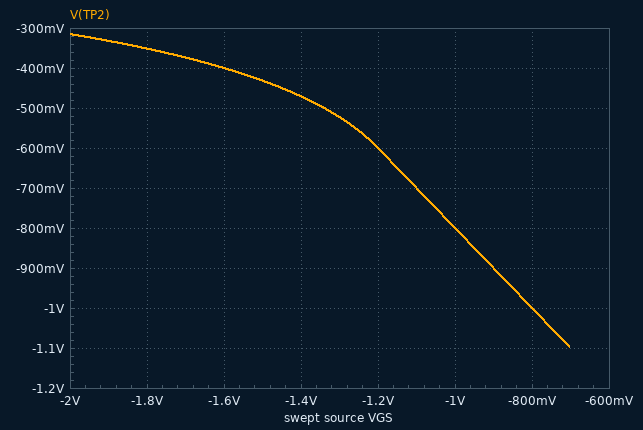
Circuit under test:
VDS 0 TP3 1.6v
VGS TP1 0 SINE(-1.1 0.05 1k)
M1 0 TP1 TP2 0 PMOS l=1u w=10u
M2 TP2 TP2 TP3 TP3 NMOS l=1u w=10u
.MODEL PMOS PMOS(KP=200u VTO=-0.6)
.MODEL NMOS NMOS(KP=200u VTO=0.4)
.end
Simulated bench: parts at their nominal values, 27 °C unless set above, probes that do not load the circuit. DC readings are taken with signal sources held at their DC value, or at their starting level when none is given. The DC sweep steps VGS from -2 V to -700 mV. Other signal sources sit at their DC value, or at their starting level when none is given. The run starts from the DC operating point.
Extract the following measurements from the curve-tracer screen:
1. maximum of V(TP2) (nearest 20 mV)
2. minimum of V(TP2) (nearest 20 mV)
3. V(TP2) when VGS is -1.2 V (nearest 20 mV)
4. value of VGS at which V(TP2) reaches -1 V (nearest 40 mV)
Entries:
-320 mV
-1.10 V
-600 mV
-800 mV
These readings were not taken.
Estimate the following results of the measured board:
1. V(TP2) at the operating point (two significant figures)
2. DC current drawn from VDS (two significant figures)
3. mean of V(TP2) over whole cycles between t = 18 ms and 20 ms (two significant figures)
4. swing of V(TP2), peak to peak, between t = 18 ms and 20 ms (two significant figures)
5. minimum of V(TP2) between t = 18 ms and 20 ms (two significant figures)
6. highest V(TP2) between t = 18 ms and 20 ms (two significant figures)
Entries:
-700 mV
250 µA
-700 mV
100 mV
-750 mV
-650 mV
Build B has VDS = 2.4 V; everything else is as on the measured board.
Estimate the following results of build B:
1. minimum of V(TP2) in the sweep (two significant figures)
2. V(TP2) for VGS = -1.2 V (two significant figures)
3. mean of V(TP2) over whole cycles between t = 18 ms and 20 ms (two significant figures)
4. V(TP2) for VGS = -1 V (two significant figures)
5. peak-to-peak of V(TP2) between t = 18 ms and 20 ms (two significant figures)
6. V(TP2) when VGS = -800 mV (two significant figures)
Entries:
-1.9 V
-1.4 V
-1.5 V
-1.6 V
100 mV
-1.8 V
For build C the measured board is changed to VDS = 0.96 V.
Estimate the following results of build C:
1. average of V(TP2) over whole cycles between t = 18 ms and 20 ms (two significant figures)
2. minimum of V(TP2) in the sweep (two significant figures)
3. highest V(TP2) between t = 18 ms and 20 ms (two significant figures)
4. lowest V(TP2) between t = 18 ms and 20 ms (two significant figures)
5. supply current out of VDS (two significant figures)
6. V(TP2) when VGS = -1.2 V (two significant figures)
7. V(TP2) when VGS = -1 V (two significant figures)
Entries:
-180 mV
-460 mV
-170 mV
-190 mV
150 µA
-160 mV
-210 mV
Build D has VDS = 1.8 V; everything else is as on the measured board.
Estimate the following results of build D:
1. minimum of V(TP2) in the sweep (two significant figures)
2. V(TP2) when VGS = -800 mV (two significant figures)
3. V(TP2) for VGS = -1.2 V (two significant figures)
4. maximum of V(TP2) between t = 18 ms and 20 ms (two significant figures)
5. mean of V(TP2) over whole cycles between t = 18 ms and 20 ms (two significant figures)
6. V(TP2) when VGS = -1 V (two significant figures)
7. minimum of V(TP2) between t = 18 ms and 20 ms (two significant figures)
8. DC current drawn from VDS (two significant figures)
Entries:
-1.3 V
-1.2 V
-800 mV
-850 mV
-900 mV
-1.0 V
-950 mV
250 µA
